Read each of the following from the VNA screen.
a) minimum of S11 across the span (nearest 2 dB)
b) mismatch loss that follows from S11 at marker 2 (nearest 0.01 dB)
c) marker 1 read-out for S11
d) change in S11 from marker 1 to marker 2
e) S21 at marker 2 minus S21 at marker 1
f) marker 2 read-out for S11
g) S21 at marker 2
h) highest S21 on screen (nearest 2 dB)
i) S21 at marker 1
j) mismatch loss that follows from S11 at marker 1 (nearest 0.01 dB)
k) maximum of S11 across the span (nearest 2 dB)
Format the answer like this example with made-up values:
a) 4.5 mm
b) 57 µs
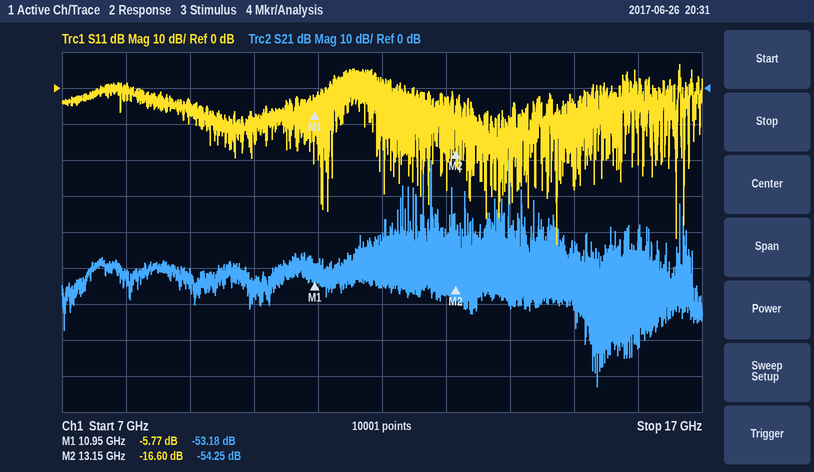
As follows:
a) -44 dB
b) 0.10 dB
c) -5.77 dB
d) -10.83 dB
e) -1.07 dB
f) -16.60 dB
g) -54.25 dB
h) -20 dB
i) -53.18 dB
j) 1.34 dB
k) 6 dB
